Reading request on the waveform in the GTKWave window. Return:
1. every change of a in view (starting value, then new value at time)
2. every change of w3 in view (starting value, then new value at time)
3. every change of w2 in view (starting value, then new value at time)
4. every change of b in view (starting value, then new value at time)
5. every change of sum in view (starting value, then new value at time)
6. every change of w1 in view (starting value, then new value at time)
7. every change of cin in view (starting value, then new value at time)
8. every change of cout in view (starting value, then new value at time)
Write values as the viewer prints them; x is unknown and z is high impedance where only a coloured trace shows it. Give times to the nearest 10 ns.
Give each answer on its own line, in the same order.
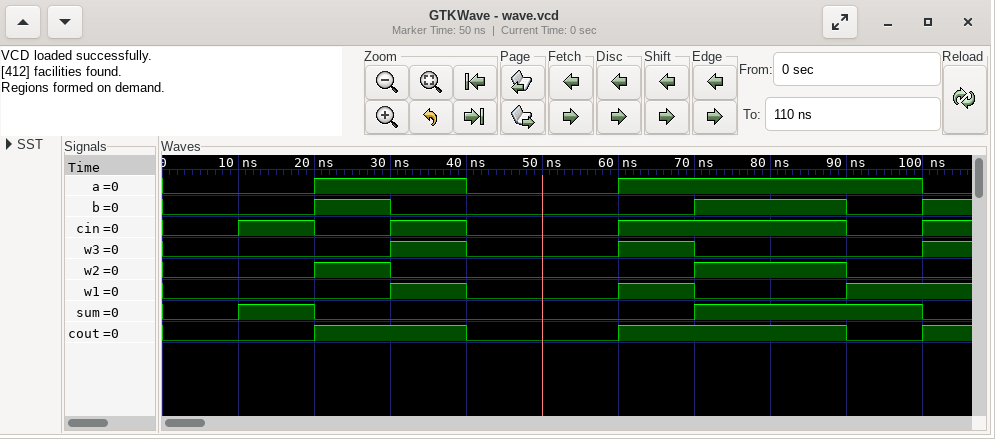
0, 1 at 20 ns, 0 at 40 ns, 1 at 60 ns, 0 at 100 ns
0, 1 at 30 ns, 0 at 40 ns, 1 at 60 ns, 0 at 70 ns, 1 at 100 ns
0, 1 at 20 ns, 0 at 30 ns, 1 at 70 ns, 0 at 90 ns
0, 1 at 20 ns, 0 at 30 ns, 1 at 70 ns, 0 at 90 ns, 1 at 100 ns
0, 1 at 10 ns, 0 at 20 ns, 1 at 70 ns, 0 at 100 ns
0, 1 at 30 ns, 0 at 40 ns, 1 at 60 ns, 0 at 70 ns, 1 at 90 ns
0, 1 at 10 ns, 0 at 20 ns, 1 at 30 ns, 0 at 40 ns, 1 at 60 ns, 0 at 90 ns, 1 at 100 ns
0, 1 at 20 ns, 0 at 40 ns, 1 at 60 ns, 0 at 90 ns, 1 at 100 ns
